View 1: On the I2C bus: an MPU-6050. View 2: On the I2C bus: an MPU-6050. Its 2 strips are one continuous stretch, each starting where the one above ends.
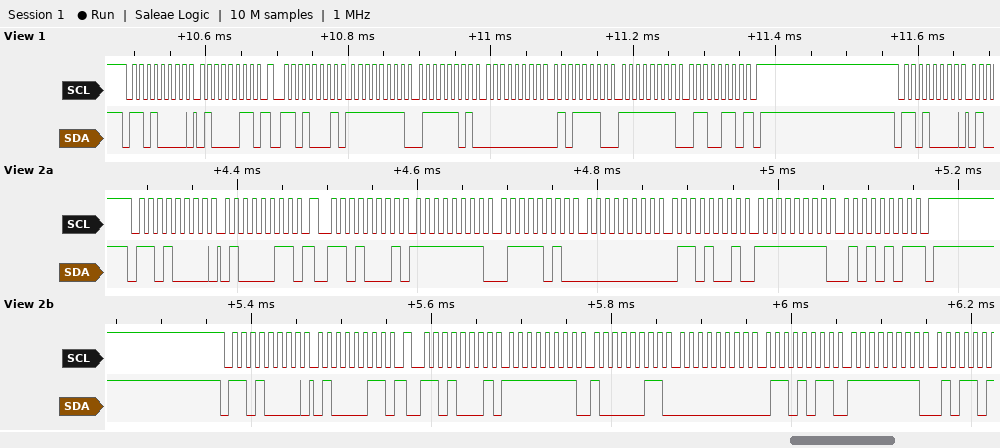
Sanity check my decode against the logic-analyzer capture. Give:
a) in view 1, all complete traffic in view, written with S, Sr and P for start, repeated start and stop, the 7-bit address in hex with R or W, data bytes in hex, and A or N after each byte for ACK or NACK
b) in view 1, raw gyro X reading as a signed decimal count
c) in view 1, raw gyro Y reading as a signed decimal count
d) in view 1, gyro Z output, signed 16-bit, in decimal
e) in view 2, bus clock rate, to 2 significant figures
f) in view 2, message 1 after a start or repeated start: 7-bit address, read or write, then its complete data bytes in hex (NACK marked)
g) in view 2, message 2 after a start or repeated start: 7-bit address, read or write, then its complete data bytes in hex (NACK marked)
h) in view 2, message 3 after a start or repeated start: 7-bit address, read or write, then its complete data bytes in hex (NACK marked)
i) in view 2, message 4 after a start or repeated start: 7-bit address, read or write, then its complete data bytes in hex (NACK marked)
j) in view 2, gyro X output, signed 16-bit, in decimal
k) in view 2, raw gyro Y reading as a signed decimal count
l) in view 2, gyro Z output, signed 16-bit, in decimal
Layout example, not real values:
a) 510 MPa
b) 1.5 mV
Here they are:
a) S 68W A 43 A Sr 68R A FF A 7D A 00 A 5E A FF A 66 N P S 68W A
b) -131
c) 94
d) -154
e) 100 kHz
f) 0x68 write: 43
g) 0x68 read: FF 7A 00 69 FF 55 NACK
h) 0x68 write: 43
i) 0x68 read: FF 83 00 6B FF
j) -134
k) 105
l) -171
